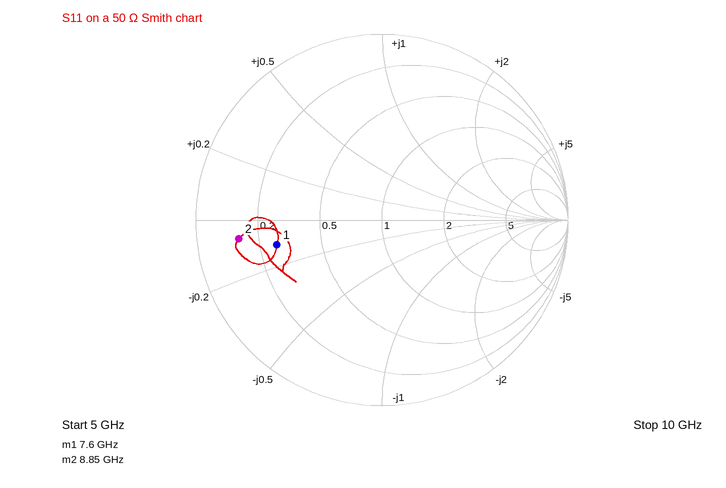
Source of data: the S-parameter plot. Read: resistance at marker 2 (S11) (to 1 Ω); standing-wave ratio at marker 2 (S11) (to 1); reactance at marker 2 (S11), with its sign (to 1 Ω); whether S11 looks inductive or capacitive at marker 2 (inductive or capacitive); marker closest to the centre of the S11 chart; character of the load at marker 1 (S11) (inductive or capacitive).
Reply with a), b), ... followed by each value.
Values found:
a) 6 Ω
b) 8
c) -3 Ω
d) capacitive
e) marker 1
f) capacitive
